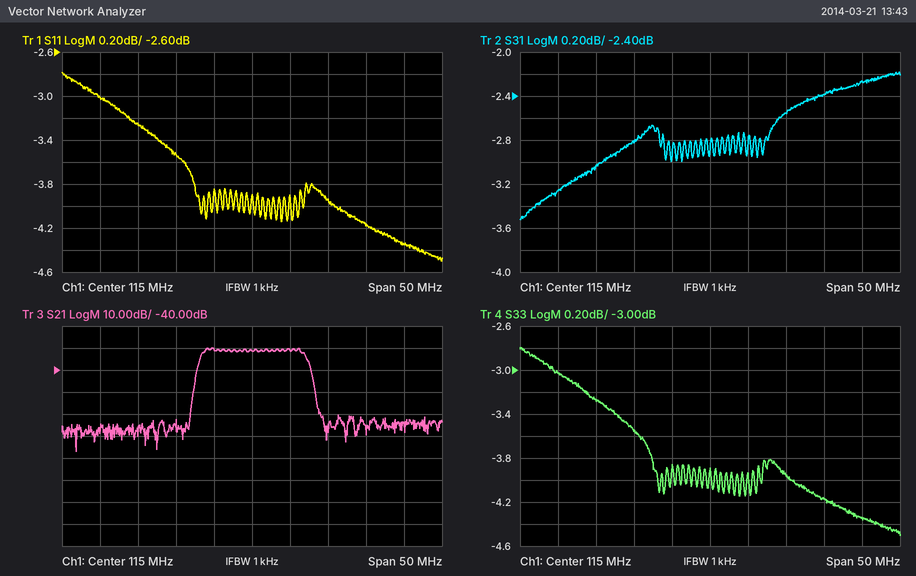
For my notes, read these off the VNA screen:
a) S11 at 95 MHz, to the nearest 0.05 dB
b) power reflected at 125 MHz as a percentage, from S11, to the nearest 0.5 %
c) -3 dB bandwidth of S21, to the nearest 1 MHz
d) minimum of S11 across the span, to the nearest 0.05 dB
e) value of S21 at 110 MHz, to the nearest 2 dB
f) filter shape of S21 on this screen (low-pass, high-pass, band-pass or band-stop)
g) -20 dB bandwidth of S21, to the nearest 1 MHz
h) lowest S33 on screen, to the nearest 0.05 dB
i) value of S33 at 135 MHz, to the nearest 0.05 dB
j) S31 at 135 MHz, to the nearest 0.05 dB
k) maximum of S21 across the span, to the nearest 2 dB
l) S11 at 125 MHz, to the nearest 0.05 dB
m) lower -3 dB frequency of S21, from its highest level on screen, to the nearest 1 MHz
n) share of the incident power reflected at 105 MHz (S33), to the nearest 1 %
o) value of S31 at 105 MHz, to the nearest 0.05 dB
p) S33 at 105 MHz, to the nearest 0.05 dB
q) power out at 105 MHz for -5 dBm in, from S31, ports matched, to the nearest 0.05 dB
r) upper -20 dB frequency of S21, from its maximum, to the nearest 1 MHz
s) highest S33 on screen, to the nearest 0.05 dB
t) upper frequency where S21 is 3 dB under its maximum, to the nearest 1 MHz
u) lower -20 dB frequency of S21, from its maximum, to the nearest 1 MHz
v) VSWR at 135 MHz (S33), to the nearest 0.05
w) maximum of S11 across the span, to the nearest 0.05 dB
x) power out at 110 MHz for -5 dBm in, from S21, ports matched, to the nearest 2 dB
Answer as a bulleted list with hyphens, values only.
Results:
- -3.00 dB
- 40.5 %
- 14 MHz
- -4.50 dB
- -30 dB
- band-pass
- 16 MHz
- -4.50 dB
- -4.35 dB
- -2.25 dB
- -30 dB
- -3.95 dB
- 108 MHz
- 44 %
- -2.80 dB
- -3.55 dB
- -7.80 dBm
- 123 MHz
- -2.80 dB
- 122 MHz
- 107 MHz
- 4.10
- -2.80 dB
- -36 dBm
